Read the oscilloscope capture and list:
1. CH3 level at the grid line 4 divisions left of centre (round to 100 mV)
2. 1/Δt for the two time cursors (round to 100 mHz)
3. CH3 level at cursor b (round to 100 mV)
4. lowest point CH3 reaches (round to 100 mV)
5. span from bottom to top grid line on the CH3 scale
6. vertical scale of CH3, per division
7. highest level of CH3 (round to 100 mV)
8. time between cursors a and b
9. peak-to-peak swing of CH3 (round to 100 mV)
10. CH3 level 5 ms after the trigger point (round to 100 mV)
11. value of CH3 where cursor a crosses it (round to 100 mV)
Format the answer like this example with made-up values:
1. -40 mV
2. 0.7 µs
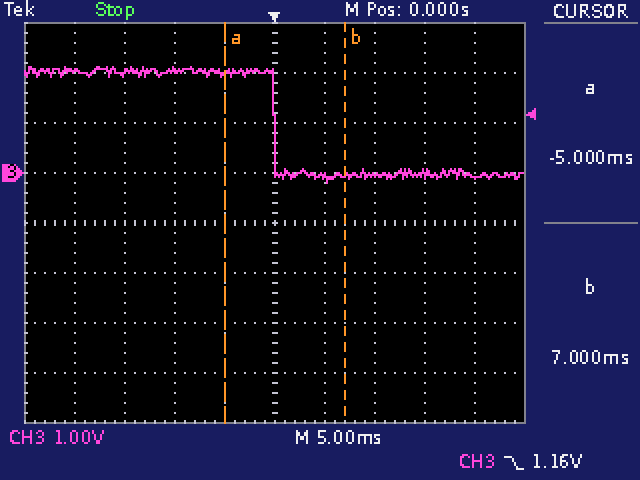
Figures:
1. 2.0 V
2. 83.3 Hz
3. -100 mV
4. -200 mV
5. 8 V
6. 1 V
7. 2.1 V
8. 12.0 ms
9. 2.3 V
10. -100 mV
11. 2.0 V
